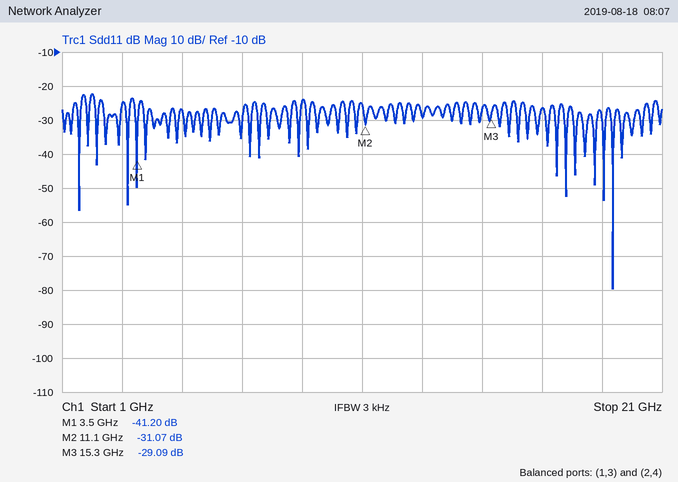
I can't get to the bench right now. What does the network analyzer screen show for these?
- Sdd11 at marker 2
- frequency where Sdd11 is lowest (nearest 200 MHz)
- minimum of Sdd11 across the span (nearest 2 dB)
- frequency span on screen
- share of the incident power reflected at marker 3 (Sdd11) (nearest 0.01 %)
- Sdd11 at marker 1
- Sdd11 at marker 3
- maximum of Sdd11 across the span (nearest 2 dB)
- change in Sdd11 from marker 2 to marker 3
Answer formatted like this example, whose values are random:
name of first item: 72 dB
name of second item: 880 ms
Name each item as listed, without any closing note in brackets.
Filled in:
Sdd11 at marker 2: -31.07 dB
frequency where Sdd11 is lowest: 19.4 GHz
minimum of Sdd11 across the span: -80 dB
frequency span on screen: 20 GHz
share of the incident power reflected at marker 3 (Sdd11): 0.12 %
Sdd11 at marker 1: -41.20 dB
Sdd11 at marker 3: -29.09 dB
maximum of Sdd11 across the span: -22 dB
change in Sdd11 from marker 2 to marker 3: 1.98 dB
